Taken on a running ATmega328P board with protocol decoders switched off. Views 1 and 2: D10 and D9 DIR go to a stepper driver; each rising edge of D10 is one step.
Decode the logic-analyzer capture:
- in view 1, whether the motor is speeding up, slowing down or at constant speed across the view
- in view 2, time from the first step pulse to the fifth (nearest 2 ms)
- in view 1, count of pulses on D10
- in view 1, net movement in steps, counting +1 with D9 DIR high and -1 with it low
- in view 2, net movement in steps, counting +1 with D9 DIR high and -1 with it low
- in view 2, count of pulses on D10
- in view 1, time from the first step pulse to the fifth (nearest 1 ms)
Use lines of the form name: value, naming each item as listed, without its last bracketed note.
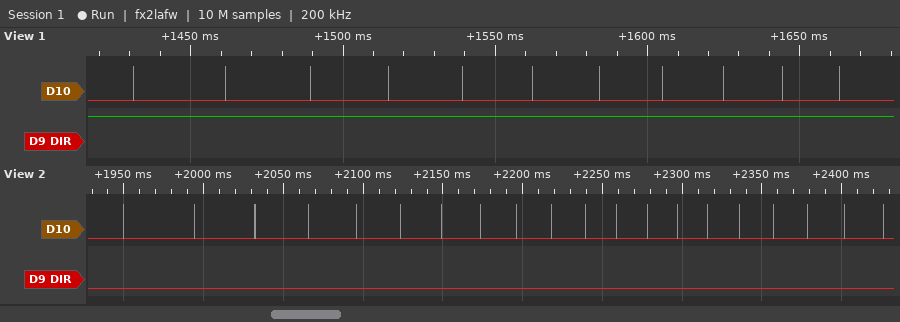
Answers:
in view 1, whether the motor is speeding up, slowing down or at constant speed across the view: speeding up
in view 2, time from the first step pulse to the fifth: 146 ms
in view 1, count of pulses on D10: 11
in view 1, net movement in steps, counting +1 with D9 DIR high and -1 with it low: +11
in view 2, net movement in steps, counting +1 with D9 DIR high and -1 with it low: -20
in view 2, count of pulses on D10: 20
in view 1, time from the first step pulse to the fifth: 108 ms
